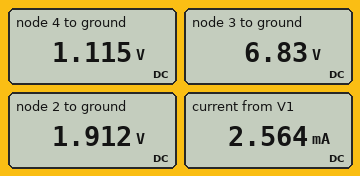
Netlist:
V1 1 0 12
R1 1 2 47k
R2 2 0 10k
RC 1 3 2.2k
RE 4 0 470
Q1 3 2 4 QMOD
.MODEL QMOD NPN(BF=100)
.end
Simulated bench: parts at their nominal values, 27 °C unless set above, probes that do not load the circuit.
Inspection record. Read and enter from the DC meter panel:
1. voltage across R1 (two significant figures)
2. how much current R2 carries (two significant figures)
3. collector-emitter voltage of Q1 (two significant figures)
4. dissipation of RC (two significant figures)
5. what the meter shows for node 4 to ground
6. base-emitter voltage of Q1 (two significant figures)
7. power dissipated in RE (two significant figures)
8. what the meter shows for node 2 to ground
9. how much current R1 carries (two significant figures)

10 V
190 µA
5.7 V
12 mW
1.115 V
800 mV
2.6 mW
1.912 V
210 µA
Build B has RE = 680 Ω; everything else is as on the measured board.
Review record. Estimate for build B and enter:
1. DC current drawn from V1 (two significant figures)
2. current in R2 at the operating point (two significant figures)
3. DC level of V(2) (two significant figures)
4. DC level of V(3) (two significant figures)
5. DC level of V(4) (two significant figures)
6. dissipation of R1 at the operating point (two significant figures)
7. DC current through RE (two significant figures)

1.9 mA
200 µA
2.0 V
8.2 V
1.2 V
2.1 mW
1.7 mA
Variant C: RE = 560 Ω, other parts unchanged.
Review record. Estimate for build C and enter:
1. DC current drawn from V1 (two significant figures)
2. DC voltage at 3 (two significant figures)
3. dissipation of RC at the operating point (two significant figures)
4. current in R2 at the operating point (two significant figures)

2.2 mA
7.5 V
9.0 mW
190 µA
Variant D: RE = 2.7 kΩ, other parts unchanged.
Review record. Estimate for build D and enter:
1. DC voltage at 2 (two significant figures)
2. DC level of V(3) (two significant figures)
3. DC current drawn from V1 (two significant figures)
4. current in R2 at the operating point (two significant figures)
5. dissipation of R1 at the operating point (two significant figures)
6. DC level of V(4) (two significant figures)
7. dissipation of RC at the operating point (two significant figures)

2.1 V
11 V
690 µA
210 µA
2.1 mW
1.3 V
510 µW
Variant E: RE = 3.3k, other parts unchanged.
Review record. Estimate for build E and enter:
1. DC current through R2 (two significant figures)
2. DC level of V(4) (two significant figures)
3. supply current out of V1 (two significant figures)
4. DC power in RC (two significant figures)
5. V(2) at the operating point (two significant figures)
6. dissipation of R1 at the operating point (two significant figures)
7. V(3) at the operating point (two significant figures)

210 µA
1.3 V
610 µA
350 µW
2.1 V
2.1 mW
11 V
